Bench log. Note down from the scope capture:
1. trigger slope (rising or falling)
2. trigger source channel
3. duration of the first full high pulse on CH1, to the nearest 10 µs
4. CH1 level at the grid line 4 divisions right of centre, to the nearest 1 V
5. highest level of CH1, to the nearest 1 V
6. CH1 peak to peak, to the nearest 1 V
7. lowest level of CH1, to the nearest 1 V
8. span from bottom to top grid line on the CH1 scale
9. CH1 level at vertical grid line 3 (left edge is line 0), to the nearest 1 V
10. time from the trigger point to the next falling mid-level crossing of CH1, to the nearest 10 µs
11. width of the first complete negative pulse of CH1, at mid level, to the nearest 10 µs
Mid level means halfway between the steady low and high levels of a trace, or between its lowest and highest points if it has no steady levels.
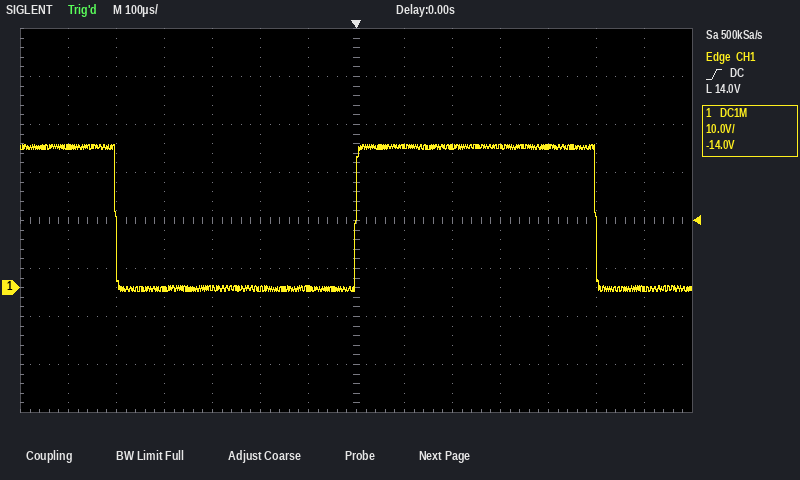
rising
CH1
500 µs
29 V
30 V
31 V
-1 V
80 V
0 V
500 µs
500 µs
